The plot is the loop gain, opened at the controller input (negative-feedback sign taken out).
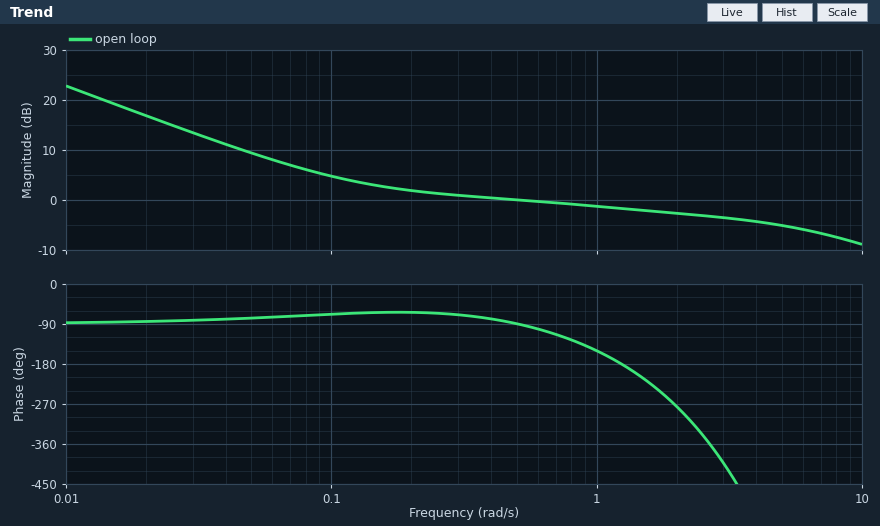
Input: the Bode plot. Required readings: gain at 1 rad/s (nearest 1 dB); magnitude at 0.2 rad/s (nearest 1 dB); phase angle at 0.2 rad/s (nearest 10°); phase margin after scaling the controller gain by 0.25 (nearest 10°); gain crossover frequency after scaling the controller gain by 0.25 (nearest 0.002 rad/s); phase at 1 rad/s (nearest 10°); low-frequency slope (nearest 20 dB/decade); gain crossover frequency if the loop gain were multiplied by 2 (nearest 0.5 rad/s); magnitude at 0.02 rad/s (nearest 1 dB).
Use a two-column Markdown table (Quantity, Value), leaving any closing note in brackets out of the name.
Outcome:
| Quantity | Value |
|---|---|
| gain at 1 rad/s | -1 dB |
| magnitude at 0.2 rad/s | 2 dB |
| phase angle at 0.2 rad/s | -60° |
| phase margin after scaling the controller gain by 0.25 | 100° |
| gain crossover frequency after scaling the controller gain by 0.25 | 0.036 rad/s |
| phase at 1 rad/s | -150° |
| low-frequency slope | -20 dB/decade |
| gain crossover frequency if the loop gain were multiplied by 2 | 6.0 rad/s |
| magnitude at 0.02 rad/s | 17 dB |
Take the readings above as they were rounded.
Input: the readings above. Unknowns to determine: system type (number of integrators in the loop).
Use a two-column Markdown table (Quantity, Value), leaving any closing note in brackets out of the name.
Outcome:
| Quantity | Value |
|---|---|
| system type | 1 |
